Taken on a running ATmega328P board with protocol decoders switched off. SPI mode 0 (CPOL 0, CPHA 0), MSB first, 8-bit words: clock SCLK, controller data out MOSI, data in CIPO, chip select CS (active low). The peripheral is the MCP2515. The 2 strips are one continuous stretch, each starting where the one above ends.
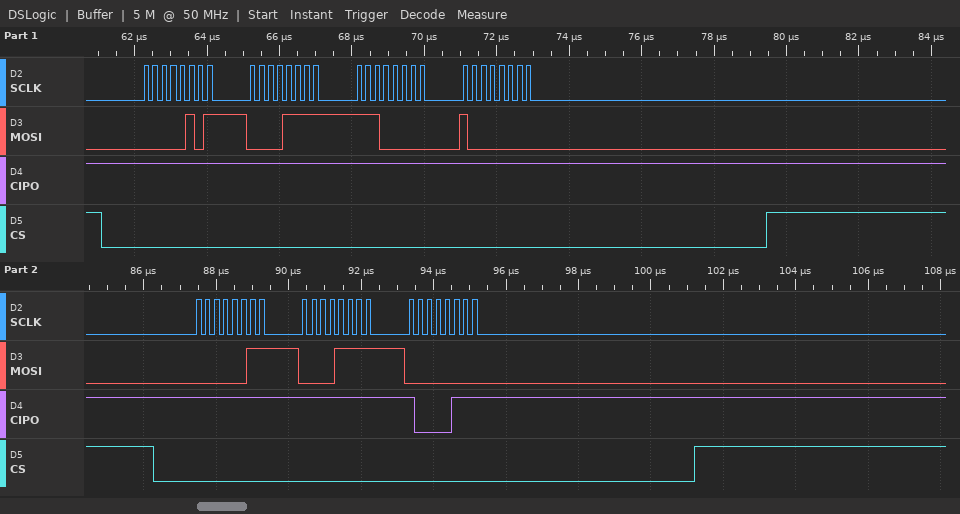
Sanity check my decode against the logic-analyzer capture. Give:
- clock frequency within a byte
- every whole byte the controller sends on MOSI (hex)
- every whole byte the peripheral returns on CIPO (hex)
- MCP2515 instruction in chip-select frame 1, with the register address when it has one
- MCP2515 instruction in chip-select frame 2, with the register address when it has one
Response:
4 MHz
05 0F E0 80 03 0F 00
FF FF FF FF FF FF 87
BIT MODIFY 0x0F
READ 0x0F
